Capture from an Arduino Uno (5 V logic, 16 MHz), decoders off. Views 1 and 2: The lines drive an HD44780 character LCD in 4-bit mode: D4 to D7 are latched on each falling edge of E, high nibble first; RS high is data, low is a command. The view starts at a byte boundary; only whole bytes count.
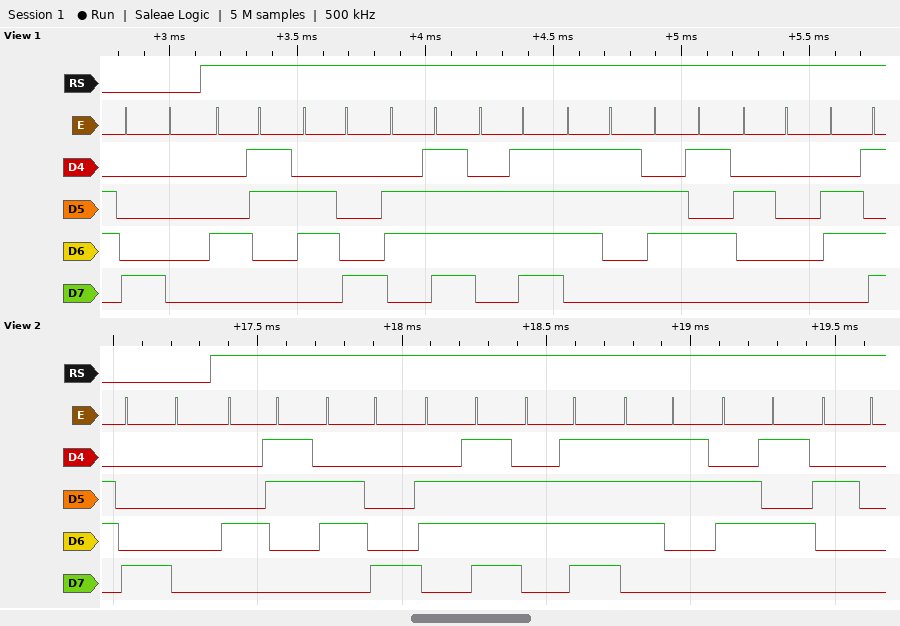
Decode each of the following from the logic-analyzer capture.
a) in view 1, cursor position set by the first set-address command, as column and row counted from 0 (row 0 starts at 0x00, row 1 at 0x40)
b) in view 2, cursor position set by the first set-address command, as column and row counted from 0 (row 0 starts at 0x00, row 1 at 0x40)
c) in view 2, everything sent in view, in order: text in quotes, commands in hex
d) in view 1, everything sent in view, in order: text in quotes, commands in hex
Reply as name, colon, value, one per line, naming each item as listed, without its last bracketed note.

in view 1, cursor position set by the first set-address command, as column and row counted from 0: column 0, row 0
in view 2, cursor position set by the first set-address command, as column and row counted from 0: column 0, row 0
in view 2, everything sent in view, in order: text in quotes, commands in hex: 0x80 "Choose "
in view 1, everything sent in view, in order: text in quotes, commands in hex: 0x80 "Choose m"
